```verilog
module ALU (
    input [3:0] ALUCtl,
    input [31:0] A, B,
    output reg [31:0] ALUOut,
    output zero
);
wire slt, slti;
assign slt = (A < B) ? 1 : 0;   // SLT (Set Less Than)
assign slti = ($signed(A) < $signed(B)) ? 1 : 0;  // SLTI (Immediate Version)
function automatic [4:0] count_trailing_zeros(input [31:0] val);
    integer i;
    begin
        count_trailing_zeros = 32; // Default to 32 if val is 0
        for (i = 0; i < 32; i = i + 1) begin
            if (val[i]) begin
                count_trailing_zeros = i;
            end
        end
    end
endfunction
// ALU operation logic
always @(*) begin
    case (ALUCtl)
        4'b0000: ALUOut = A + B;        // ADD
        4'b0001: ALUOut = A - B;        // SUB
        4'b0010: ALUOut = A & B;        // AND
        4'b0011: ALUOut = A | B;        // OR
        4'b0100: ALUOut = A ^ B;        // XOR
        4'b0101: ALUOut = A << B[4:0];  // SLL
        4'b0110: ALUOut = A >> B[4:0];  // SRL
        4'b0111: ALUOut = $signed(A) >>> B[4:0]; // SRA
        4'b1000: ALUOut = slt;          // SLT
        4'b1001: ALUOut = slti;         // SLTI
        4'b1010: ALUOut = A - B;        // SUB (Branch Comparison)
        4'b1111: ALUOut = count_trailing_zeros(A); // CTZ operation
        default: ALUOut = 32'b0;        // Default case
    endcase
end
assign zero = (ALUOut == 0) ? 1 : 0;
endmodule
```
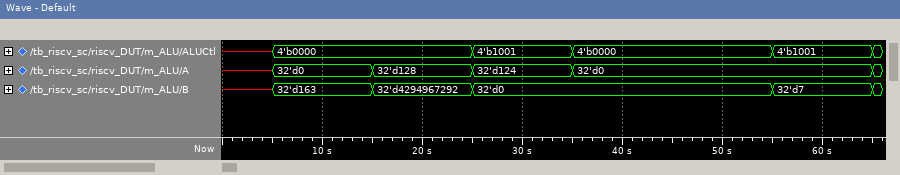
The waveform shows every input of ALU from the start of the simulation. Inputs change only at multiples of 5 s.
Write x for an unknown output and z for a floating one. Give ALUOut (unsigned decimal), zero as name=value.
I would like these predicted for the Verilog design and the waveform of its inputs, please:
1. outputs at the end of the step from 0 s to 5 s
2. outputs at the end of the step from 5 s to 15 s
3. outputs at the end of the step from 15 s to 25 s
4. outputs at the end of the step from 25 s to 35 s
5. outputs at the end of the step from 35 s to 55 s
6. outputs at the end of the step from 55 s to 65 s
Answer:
ALUOut=0, zero=1
ALUOut=163, zero=0
ALUOut=124, zero=0
ALUOut=0, zero=1
ALUOut=0, zero=1
ALUOut=1, zero=0
